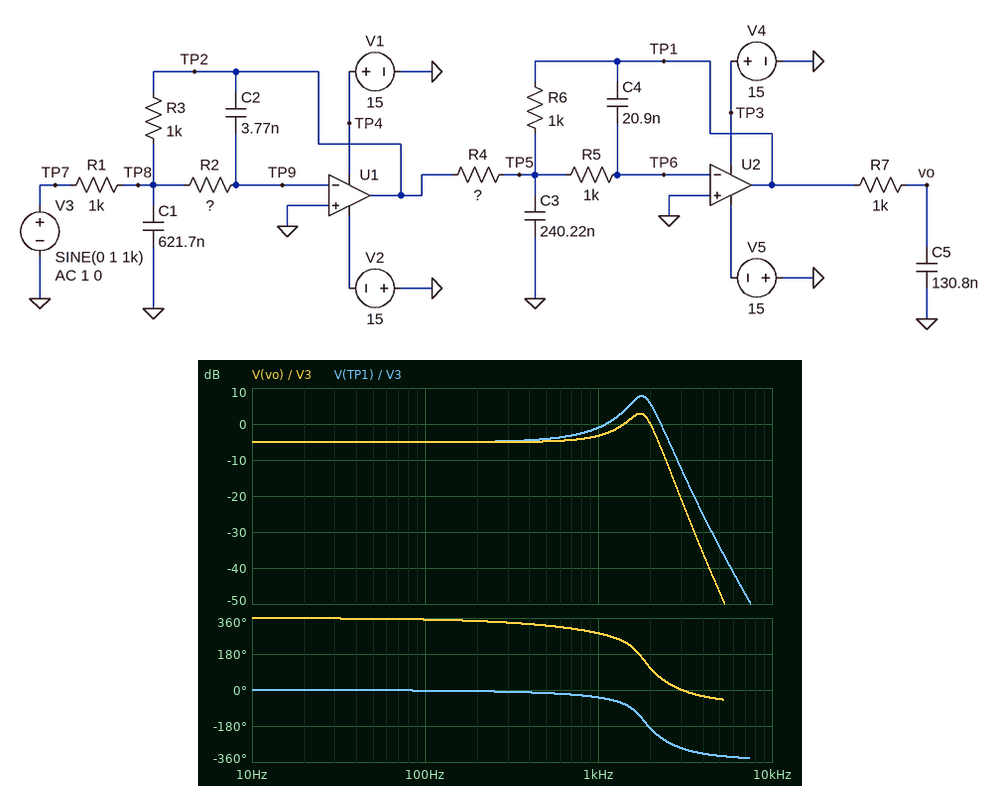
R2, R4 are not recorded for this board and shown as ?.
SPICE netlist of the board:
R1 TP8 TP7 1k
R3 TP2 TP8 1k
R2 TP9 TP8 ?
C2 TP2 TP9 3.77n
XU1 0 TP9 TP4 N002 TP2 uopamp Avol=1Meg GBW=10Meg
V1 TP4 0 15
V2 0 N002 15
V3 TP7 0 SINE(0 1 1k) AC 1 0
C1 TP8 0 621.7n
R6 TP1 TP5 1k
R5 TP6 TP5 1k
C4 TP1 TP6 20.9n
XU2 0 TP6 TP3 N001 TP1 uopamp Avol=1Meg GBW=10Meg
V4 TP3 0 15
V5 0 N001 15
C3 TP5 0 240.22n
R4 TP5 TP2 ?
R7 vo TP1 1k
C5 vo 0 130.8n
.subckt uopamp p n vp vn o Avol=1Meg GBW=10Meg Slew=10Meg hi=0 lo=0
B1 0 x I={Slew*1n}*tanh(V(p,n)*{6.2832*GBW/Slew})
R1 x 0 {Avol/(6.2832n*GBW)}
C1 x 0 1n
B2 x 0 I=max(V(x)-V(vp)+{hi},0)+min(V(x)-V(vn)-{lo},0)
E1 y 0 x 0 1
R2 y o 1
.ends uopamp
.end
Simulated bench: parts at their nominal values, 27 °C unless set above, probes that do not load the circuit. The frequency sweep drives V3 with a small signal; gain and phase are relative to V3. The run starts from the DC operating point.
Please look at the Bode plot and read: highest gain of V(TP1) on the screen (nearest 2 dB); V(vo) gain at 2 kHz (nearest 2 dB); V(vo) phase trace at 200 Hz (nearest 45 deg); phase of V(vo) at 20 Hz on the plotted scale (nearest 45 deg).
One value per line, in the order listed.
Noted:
8 dB
0 dB
360 deg
360 deg
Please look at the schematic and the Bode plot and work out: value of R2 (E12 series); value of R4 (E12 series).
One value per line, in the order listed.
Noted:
3.3 kΩ
1.8 kΩ
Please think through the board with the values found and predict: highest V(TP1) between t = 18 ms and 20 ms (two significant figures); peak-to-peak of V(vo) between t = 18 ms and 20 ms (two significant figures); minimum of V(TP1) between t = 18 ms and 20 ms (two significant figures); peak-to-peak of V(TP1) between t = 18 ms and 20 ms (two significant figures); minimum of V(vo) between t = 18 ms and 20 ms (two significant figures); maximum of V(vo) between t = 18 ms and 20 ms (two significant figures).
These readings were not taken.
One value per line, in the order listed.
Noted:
890 mV
1.4 V
-890 mV
1.8 V
-690 mV
690 mV
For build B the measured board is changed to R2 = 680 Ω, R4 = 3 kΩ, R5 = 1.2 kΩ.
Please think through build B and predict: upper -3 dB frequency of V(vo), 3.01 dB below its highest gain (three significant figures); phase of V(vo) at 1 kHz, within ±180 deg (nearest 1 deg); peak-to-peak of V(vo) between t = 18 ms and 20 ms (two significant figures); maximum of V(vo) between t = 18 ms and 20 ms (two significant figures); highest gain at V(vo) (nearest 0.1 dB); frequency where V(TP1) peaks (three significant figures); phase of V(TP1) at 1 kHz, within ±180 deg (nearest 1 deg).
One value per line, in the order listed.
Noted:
2.43 kHz
-67 deg
660 mV
330 mV
-8.9 dB
1.95 kHz
-28 deg
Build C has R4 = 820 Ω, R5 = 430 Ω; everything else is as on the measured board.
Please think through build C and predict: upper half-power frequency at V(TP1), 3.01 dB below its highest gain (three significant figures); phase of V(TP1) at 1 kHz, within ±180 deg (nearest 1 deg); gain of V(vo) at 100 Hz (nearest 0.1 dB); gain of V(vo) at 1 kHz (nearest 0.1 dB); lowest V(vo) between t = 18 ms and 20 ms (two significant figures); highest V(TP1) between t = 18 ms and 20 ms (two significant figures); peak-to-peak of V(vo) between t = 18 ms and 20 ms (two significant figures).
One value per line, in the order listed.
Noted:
2.06 kHz
-30 deg
1.7 dB
2.8 dB
-1.4 V
1.8 V
2.8 V
